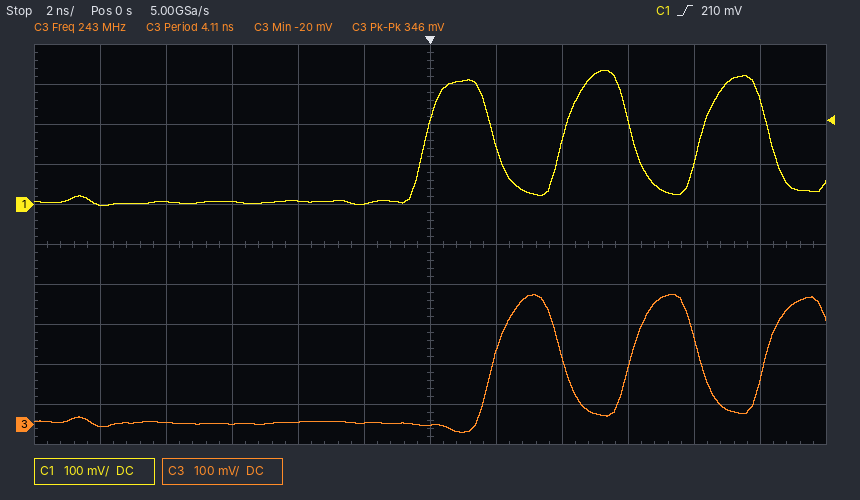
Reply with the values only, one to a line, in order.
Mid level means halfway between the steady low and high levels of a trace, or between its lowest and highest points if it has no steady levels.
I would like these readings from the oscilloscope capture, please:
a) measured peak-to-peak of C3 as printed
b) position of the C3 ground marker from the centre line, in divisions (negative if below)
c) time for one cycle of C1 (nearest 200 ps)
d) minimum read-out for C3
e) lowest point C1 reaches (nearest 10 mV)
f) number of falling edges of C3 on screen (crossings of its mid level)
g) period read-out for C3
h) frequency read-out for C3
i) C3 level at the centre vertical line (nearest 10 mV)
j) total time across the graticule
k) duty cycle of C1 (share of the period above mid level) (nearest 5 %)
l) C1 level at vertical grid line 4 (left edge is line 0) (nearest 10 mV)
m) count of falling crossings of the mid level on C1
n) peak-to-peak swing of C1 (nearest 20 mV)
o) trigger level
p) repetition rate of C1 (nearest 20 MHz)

346 mV
-4.5 div
4.2 ns
-20 mV
0 mV
2
4.11 ns
243 MHz
0 mV
24 ns
50 %
10 mV
3
340 mV
210 mV
240 MHz
